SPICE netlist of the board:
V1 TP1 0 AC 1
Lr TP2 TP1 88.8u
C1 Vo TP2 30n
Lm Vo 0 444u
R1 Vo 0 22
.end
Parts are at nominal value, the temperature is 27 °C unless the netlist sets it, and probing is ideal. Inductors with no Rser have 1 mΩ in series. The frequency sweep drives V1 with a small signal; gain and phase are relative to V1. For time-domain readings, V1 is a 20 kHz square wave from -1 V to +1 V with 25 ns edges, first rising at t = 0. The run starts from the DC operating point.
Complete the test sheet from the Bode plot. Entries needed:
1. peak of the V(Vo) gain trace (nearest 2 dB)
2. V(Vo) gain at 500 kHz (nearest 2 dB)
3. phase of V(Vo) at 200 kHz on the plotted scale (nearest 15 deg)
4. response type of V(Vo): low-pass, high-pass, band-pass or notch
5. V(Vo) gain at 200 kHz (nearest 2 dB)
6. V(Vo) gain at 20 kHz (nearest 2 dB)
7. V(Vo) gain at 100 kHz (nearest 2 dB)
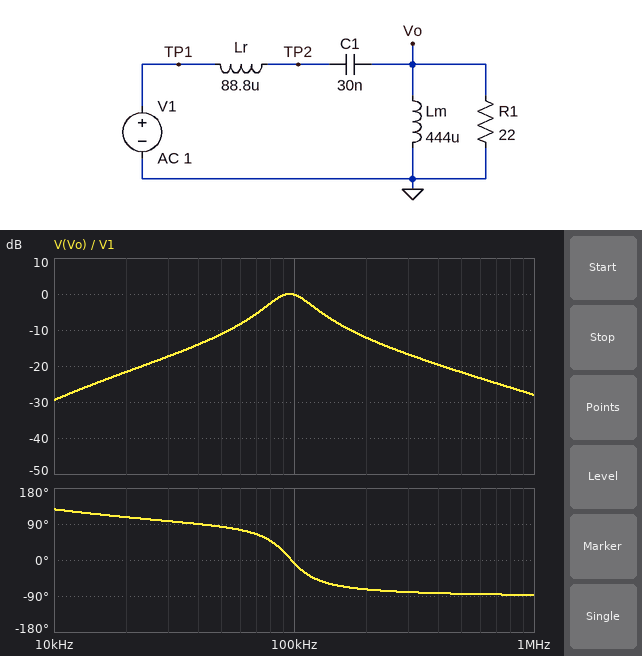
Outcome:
0 dB
-22 dB
-75 deg
band-pass
-12 dB
-22 dB
0 dB
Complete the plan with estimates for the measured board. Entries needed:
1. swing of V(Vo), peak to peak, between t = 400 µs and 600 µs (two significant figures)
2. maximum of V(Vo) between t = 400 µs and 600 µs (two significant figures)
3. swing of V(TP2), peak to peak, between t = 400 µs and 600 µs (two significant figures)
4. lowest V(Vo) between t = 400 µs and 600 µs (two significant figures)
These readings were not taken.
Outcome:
1.2 V
600 mV
4.3 V
-600 mV
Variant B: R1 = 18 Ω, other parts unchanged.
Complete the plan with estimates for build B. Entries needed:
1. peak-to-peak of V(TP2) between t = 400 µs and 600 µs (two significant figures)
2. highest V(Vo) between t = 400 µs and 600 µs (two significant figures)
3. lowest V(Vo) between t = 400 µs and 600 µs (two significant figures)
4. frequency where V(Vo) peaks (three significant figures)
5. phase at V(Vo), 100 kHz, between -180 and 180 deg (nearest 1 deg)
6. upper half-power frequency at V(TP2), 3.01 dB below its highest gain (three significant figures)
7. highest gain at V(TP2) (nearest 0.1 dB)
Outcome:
4.6 V
530 mV
-530 mV
96.4 kHz
-9 deg
109 kHz
10.1 dB
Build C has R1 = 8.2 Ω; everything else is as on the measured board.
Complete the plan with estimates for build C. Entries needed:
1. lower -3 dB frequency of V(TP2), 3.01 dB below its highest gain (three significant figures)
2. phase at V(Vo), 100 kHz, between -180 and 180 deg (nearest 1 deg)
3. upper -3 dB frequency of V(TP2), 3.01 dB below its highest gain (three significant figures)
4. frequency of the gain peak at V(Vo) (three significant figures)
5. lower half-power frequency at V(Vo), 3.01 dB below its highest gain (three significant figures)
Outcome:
89.1 kHz
-18 deg
104 kHz
97.3 kHz
90.2 kHz
